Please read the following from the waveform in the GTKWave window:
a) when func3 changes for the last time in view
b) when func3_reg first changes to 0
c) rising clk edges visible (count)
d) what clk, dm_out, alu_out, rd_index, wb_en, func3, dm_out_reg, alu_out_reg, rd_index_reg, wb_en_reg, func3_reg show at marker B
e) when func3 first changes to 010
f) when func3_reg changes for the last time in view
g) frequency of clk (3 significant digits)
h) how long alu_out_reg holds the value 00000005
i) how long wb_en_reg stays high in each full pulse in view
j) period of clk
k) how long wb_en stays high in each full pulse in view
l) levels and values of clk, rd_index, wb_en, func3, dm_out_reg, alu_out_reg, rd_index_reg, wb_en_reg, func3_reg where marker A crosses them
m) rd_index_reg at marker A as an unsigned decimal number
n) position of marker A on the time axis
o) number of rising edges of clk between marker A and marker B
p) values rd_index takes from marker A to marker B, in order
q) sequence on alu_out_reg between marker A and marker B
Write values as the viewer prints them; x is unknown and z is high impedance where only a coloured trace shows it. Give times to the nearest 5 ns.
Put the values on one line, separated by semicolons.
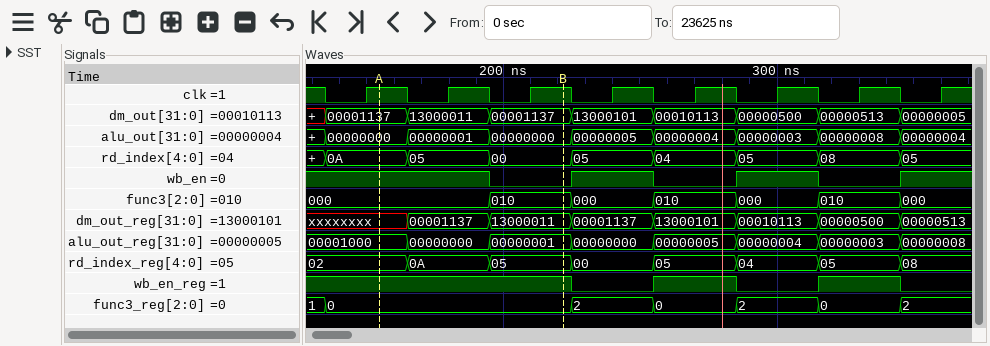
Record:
345 ns; 135 ns; 8; clk=1, dm_out=00001137, alu_out=00000000, rd_index=00, wb_en=0, func3=010, dm_out_reg=13000011, alu_out_reg=00000001, rd_index_reg=05, wb_en_reg=1, func3_reg=0; 195 ns; 345 ns; 33.3 MHz; 30 ns; 30 ns, 30 ns; 30 ns; 30 ns, 30 ns; clk=1, rd_index=0A, wb_en=1, func3=000, dm_out_reg=xxxxxxxx, alu_out_reg=00001000, rd_index_reg=02, wb_en_reg=1, func3_reg=0; 2; 155 ns; 2; 0A, 05, 00; 00001000, 00000000, 00000001
